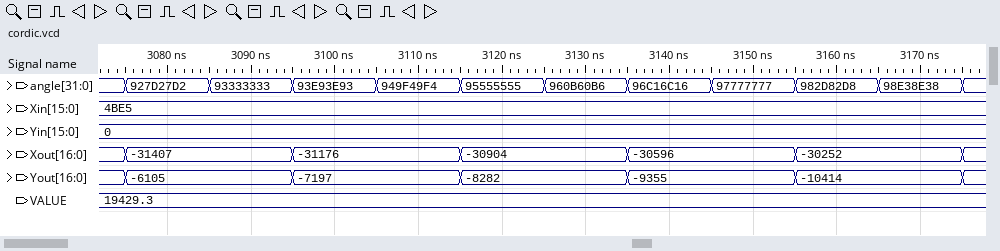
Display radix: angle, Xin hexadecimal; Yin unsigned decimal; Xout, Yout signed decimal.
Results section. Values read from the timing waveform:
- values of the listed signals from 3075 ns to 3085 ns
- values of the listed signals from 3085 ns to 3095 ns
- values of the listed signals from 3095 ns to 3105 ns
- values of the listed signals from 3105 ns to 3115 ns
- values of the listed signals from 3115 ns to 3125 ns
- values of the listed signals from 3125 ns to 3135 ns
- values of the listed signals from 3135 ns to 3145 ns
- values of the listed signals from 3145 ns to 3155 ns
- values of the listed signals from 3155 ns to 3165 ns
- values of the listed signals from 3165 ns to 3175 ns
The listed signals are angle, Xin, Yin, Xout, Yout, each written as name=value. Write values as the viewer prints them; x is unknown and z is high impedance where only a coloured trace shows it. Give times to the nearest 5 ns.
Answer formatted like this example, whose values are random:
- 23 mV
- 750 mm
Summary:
- angle=927D27D2, Xin=4BE5, Yin=0, Xout=-31407, Yout=-6105
- angle=93333333, Xin=4BE5, Yin=0, Xout=-31407, Yout=-6105
- angle=93E93E93, Xin=4BE5, Yin=0, Xout=-31176, Yout=-7197
- angle=949F49F4, Xin=4BE5, Yin=0, Xout=-31176, Yout=-7197
- angle=95555555, Xin=4BE5, Yin=0, Xout=-30904, Yout=-8282
- angle=960B60B6, Xin=4BE5, Yin=0, Xout=-30904, Yout=-8282
- angle=96C16C16, Xin=4BE5, Yin=0, Xout=-30596, Yout=-9355
- angle=97777777, Xin=4BE5, Yin=0, Xout=-30596, Yout=-9355
- angle=982D82D8, Xin=4BE5, Yin=0, Xout=-30252, Yout=-10414
- angle=98E38E38, Xin=4BE5, Yin=0, Xout=-30252, Yout=-10414
